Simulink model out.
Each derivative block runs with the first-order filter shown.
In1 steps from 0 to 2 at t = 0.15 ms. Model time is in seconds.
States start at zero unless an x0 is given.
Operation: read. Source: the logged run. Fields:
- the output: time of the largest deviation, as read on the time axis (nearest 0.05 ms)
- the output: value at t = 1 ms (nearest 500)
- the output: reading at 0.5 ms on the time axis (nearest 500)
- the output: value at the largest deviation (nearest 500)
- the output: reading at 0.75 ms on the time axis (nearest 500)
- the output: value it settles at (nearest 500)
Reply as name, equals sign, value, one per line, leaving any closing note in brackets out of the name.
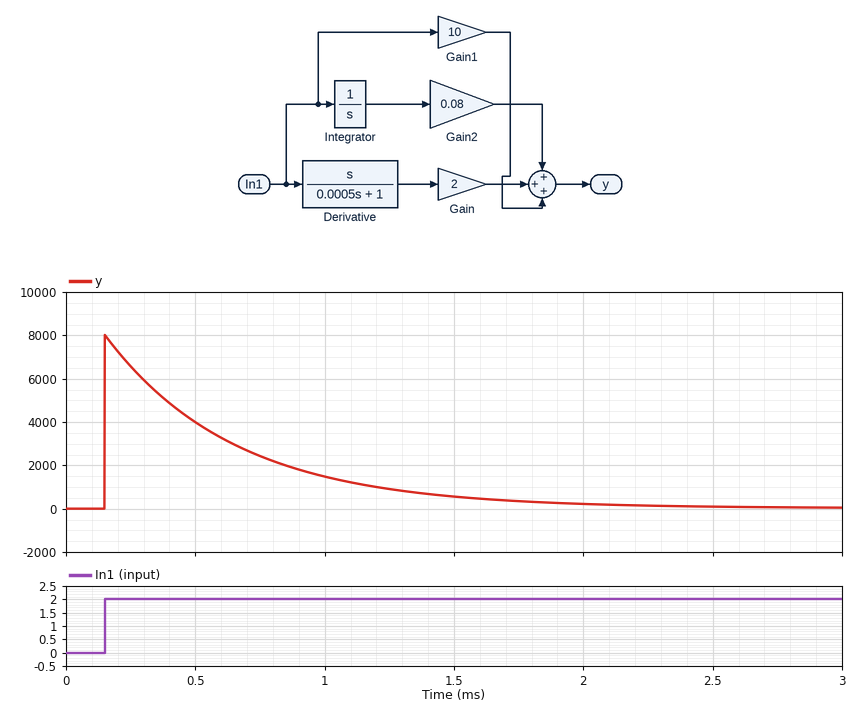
the output: time of the largest deviation, as read on the time axis = 0.15 ms
the output: value at t = 1 ms = 1500
the output: reading at 0.5 ms on the time axis = 4000
the output: value at the largest deviation = 8000
the output: reading at 0.75 ms on the time axis = 2500
the output: value it settles at = 0
